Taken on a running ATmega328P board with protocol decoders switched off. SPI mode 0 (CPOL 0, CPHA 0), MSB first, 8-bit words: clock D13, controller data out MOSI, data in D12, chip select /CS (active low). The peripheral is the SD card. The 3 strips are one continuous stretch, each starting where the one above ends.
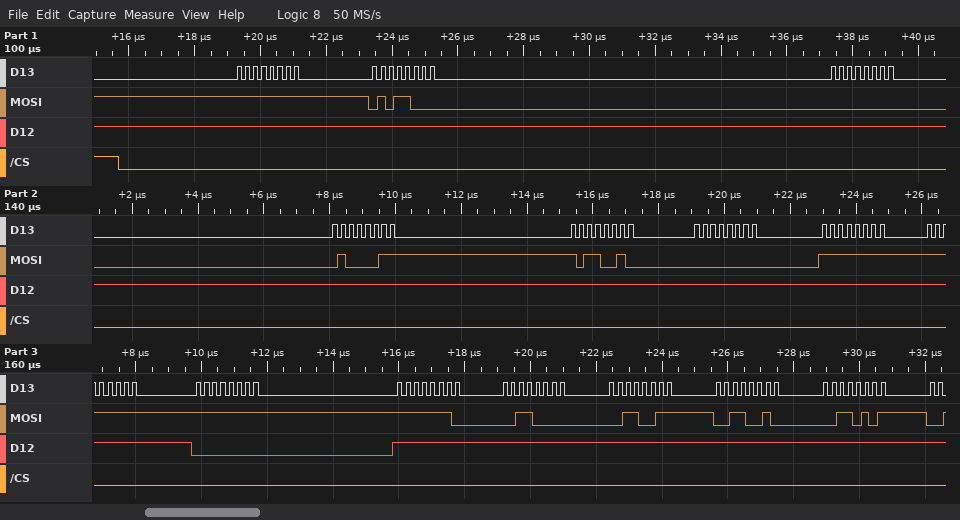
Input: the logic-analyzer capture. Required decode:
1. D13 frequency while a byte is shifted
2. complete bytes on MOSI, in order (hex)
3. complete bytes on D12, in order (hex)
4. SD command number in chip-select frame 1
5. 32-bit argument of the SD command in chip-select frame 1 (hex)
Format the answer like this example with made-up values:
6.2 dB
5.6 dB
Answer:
4 MHz
FF 58 00 43 B2 00 FF FF FF FE 30 33 32 35
FF FF FF FF FF FF FF FF 00 FF FF FF FF FF
CMD24
0x0043B200
